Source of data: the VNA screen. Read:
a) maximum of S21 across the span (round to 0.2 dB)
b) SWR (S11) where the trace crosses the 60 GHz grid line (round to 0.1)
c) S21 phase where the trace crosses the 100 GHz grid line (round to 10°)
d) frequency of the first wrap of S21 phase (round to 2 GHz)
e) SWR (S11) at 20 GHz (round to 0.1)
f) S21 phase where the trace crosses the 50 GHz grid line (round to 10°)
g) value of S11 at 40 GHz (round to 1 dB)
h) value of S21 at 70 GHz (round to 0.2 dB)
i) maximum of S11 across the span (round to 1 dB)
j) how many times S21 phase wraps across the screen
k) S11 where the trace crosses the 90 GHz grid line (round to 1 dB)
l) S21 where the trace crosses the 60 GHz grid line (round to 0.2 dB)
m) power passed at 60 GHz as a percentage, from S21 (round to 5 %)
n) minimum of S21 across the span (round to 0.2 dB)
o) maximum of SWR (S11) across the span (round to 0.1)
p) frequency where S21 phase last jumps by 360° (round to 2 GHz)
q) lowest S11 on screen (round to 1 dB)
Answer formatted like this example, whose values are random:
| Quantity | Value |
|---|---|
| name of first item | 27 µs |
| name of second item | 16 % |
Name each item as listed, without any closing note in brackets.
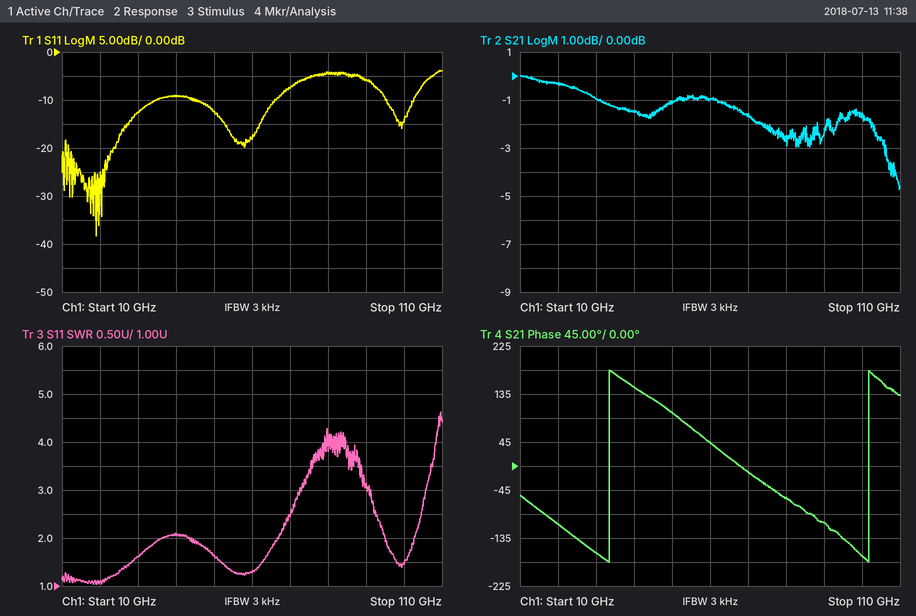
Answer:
| Quantity | Value |
|---|---|
| maximum of S21 across the span | 0.0 dB |
| SWR (S11) where the trace crosses the 60 GHz grid line | 1.3 |
| S21 phase where the trace crosses the 100 GHz grid line | -170° |
| frequency of the first wrap of S21 phase | 34 GHz |
| SWR (S11) at 20 GHz | 1.1 |
| S21 phase where the trace crosses the 50 GHz grid line | 100° |
| value of S11 at 40 GHz | -9 dB |
| value of S21 at 70 GHz | -1.6 dB |
| maximum of S11 across the span | -4 dB |
| how many times S21 phase wraps across the screen | 2 |
| S11 where the trace crosses the 90 GHz grid line | -6 dB |
| S21 where the trace crosses the 60 GHz grid line | -1.0 dB |
| power passed at 60 GHz as a percentage, from S21 | 80 % |
| minimum of S21 across the span | -4.8 dB |
| maximum of SWR (S11) across the span | 4.6 |
| frequency where S21 phase last jumps by 360° | 102 GHz |
| lowest S11 on screen | -38 dB |
